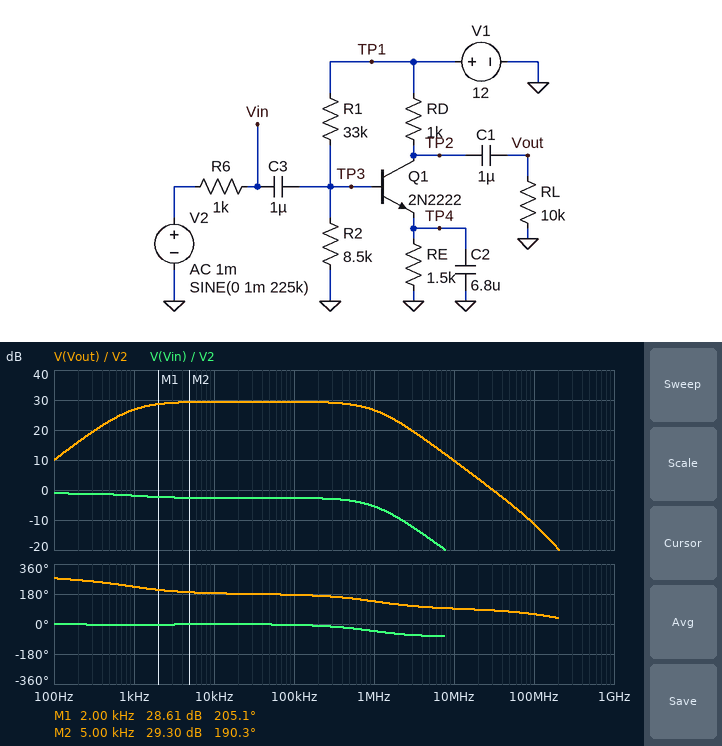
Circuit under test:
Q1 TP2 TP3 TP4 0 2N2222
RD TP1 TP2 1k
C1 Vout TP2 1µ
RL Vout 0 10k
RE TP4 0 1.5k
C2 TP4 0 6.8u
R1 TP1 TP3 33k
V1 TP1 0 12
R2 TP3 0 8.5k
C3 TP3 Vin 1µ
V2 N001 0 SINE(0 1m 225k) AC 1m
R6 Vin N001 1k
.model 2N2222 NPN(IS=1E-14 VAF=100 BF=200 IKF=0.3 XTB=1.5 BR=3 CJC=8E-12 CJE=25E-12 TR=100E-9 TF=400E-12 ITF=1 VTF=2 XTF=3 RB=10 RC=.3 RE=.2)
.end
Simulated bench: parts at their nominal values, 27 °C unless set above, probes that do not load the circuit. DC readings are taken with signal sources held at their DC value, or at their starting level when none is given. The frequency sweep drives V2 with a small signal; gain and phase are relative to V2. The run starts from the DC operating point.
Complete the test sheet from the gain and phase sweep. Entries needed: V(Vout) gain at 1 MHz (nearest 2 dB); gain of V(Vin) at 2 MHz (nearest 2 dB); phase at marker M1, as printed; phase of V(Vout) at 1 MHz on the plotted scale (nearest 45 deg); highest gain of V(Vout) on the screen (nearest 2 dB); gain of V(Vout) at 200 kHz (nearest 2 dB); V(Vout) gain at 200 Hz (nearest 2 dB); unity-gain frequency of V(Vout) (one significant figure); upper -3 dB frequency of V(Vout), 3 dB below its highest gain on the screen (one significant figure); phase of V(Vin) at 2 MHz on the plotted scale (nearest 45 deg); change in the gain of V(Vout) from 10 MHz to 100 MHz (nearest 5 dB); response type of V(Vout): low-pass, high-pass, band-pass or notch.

26 dB
-10 dB
205.1 deg
135 deg
30 dB
30 dB
16 dB
30 MHz
1 MHz
-45 deg
-20 dB
band-pass
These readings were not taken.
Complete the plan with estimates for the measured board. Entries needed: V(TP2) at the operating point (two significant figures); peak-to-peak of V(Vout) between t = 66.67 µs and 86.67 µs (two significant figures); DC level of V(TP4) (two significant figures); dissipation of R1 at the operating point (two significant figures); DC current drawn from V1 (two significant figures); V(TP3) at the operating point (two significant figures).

11 V
58 mV
1.8 V
2.8 mW
1.5 mA
2.4 V
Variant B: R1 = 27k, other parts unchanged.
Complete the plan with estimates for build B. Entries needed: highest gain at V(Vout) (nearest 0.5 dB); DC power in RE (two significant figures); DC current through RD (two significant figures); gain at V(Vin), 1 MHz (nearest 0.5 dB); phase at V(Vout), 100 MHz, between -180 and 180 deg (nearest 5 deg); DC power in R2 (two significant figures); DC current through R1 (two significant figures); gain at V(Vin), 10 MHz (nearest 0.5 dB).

31.0 dB
3.1 mW
1.4 mA
-6.5 dB
60 deg
940 µW
340 µA
-23.5 dB
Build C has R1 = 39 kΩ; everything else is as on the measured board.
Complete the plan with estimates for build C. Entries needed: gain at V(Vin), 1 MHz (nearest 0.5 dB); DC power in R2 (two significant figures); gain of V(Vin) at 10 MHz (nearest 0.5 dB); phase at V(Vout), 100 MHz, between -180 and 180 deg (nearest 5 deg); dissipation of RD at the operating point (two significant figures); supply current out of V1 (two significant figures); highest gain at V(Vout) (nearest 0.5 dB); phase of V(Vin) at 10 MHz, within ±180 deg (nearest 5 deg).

-4.5 dB
530 µW
-20.5 dB
55 deg
940 µW
1.2 mA
28.0 dB
-70 deg
